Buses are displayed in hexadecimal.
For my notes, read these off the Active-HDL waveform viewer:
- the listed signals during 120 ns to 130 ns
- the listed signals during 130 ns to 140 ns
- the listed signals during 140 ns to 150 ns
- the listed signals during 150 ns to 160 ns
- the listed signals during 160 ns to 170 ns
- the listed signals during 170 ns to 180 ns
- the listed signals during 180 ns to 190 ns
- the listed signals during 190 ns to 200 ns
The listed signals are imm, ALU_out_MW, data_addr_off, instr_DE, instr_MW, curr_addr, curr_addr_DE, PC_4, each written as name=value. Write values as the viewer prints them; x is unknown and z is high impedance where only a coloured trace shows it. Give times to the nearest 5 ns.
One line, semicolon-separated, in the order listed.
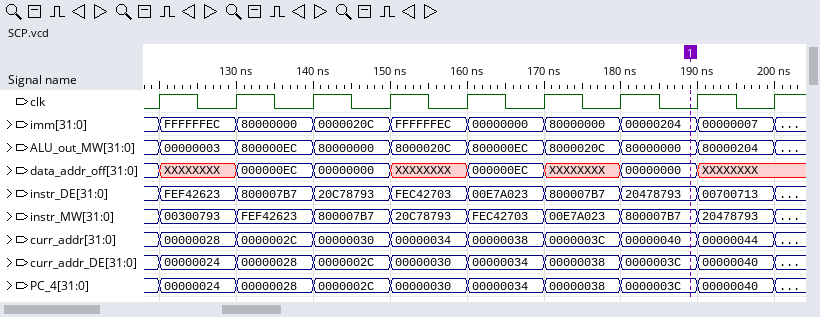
imm=FFFFFFEC, ALU_out_MW=00000003, data_addr_off=XXXXXXXX, instr_DE=FEF42623, instr_MW=00300793, curr_addr=00000028, curr_addr_DE=00000024, PC_4=00000024; imm=80000000, ALU_out_MW=800000EC, data_addr_off=000000EC, instr_DE=800007B7, instr_MW=FEF42623, curr_addr=0000002C, curr_addr_DE=00000028, PC_4=00000028; imm=0000020C, ALU_out_MW=80000000, data_addr_off=00000000, instr_DE=20C78793, instr_MW=800007B7, curr_addr=00000030, curr_addr_DE=0000002C, PC_4=0000002C; imm=FFFFFFEC, ALU_out_MW=8000020C, data_addr_off=XXXXXXXX, instr_DE=FEC42703, instr_MW=20C78793, curr_addr=00000034, curr_addr_DE=00000030, PC_4=00000030; imm=00000000, ALU_out_MW=800000EC, data_addr_off=000000EC, instr_DE=00E7A023, instr_MW=FEC42703, curr_addr=00000038, curr_addr_DE=00000034, PC_4=00000034; imm=80000000, ALU_out_MW=8000020C, data_addr_off=XXXXXXXX, instr_DE=800007B7, instr_MW=00E7A023, curr_addr=0000003C, curr_addr_DE=00000038, PC_4=00000038; imm=00000204, ALU_out_MW=80000000, data_addr_off=00000000, instr_DE=20478793, instr_MW=800007B7, curr_addr=00000040, curr_addr_DE=0000003C, PC_4=0000003C; imm=00000007, ALU_out_MW=80000204, data_addr_off=XXXXXXXX, instr_DE=00700713, instr_MW=20478793, curr_addr=00000044, curr_addr_DE=00000040, PC_4=00000040
